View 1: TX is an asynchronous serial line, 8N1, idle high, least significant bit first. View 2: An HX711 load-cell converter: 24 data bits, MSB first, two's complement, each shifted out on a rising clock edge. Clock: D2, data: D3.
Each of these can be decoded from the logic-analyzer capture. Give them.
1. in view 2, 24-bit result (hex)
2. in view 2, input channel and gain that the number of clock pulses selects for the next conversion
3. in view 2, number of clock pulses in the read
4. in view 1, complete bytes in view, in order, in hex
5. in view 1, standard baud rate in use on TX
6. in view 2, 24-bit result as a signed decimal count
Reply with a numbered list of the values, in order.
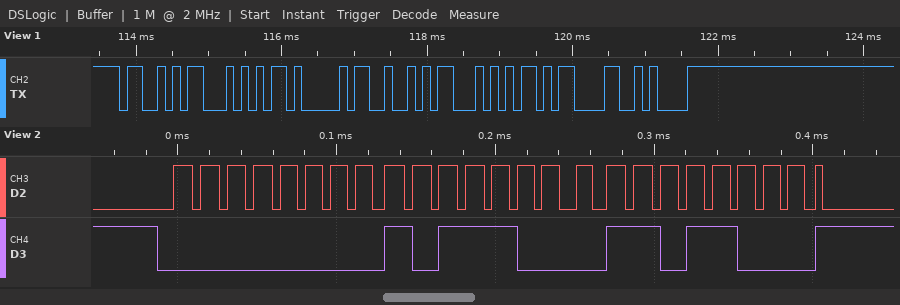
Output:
1. 0x00B8D8
2. channel A, gain 128
3. 25
4. 53 54 41 52 54 0D 0A
5. 9600 baud
6. 47320
